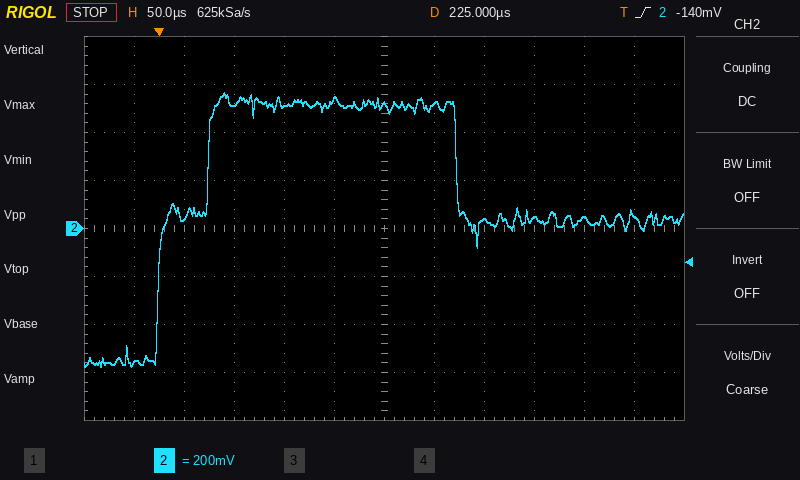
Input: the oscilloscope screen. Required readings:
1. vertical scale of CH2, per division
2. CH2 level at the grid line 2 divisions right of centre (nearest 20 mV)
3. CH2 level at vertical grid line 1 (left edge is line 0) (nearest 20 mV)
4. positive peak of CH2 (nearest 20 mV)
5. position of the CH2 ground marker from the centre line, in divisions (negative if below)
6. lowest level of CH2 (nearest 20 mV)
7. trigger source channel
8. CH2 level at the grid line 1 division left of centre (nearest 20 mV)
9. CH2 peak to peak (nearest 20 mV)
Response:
200 mV
40 mV
-560 mV
560 mV
0.0 div
-580 mV
CH2
540 mV
1.14 V
